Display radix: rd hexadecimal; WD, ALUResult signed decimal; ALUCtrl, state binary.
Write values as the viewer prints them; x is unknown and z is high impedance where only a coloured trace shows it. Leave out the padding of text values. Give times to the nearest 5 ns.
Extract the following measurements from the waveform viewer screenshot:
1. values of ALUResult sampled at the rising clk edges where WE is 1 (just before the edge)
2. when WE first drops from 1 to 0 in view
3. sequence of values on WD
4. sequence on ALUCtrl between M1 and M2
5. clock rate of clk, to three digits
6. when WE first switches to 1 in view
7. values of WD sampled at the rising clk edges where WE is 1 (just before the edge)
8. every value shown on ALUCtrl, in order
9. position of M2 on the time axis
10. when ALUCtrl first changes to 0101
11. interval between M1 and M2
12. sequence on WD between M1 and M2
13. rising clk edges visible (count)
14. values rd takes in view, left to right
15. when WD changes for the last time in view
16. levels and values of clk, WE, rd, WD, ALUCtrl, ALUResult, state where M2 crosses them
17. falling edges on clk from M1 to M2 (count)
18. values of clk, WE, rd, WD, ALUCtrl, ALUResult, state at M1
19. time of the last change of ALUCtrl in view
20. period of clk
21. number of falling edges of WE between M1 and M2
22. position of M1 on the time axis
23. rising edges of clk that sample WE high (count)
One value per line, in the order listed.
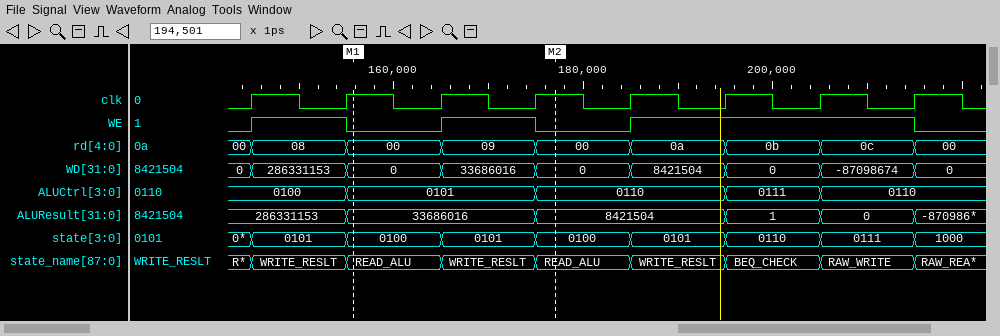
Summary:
286331153, 33686016, 8421504, 1, 0
155 ns
0, 286331153, 0, 33686016, 0, 8421504, 0, -87098674, 0
0101, 0110
100 MHz
145 ns
286331153, 33686016, 8421504, 0, -87098674
0100, 0101, 0110, 0111, 0110
175 ns
155 ns
20 ns
0, 33686016, 0
8
00, 08, 00, 09, 00, 0a, 0b, 0c, 00
215 ns
clk=1, WE=0, rd=00, WD=0, ALUCtrl=0110, ALUResult=8421504, state=0100
2
clk=1, WE=0, rd=00, WD=0, ALUCtrl=0101, ALUResult=33686016, state=0100
205 ns
10 ns
1
155 ns
5
